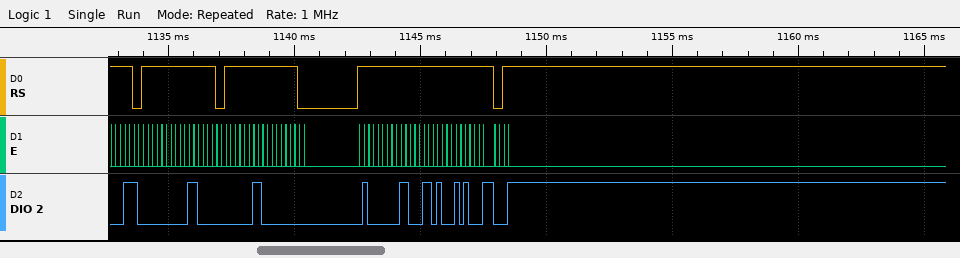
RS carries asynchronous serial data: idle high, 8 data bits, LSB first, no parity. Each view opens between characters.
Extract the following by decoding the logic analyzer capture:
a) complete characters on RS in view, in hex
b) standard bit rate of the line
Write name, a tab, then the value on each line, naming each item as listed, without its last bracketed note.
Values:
complete characters on RS in view, in hex	7F, E0, FF
standard bit rate of the line	2400 baud
